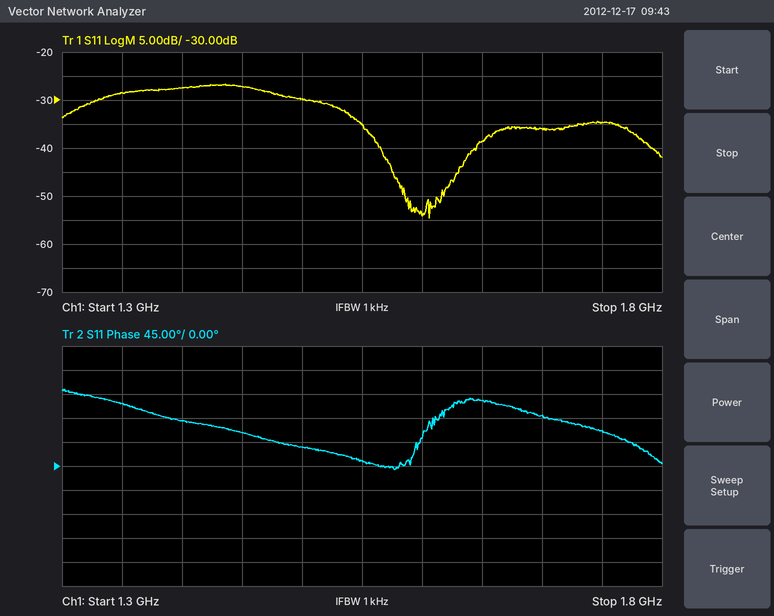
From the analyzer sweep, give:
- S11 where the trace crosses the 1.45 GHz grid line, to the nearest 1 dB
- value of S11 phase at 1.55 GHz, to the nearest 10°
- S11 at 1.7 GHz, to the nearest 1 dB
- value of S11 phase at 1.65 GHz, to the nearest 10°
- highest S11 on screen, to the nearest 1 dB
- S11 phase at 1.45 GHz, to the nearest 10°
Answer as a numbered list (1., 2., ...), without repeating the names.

1. -27 dB
2. 10°
3. -36 dB
4. 120°
5. -27 dB
6. 60°
